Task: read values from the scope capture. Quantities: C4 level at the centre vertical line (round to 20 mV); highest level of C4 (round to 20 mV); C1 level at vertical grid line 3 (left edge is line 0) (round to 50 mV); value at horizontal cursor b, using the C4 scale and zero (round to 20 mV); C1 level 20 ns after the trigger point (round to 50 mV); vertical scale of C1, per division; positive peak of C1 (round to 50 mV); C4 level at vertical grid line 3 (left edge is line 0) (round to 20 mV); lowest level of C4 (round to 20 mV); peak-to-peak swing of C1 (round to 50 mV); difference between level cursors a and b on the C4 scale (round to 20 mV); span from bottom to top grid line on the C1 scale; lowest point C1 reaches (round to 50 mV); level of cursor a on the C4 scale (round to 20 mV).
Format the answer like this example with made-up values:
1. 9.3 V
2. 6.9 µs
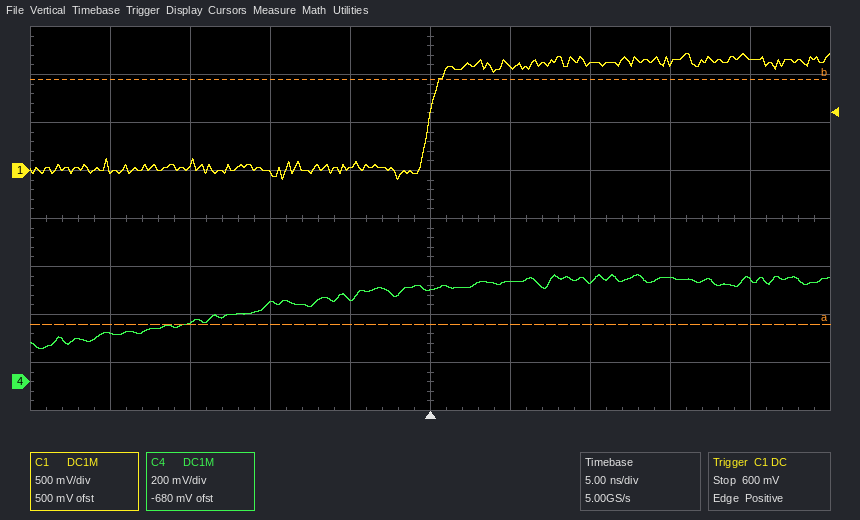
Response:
1. 380 mV
2. 440 mV
3. -50 mV
4. 1.26 V
5. 1.15 V
6. 500 mV
7. 1.20 V
8. 320 mV
9. 140 mV
10. 1.30 V
11. 1.02 V
12. 4 V
13. -100 mV
14. 240 mV
